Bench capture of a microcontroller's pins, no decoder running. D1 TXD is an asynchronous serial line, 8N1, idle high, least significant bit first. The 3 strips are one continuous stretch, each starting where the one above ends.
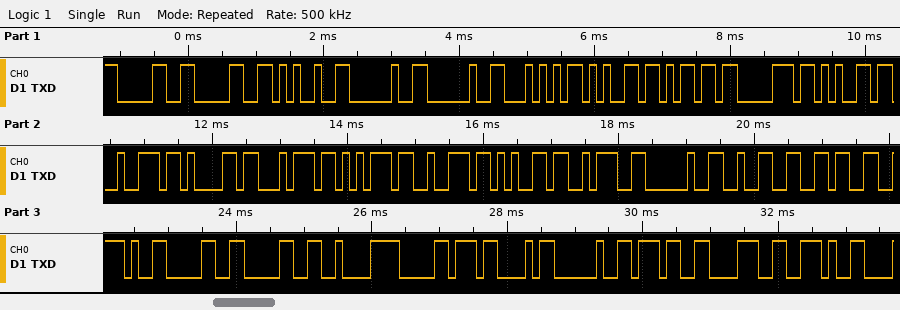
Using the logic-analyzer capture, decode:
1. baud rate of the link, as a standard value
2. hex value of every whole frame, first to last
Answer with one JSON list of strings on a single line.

["9600 baud", "0x30 0x30 0x25 0x20 0x20 0x54 0x65 0x6D 0x70 0x65 0x72 0x61 0x74 0x75 0x72 0x65 0x3A 0x20 0x32 0x36 0x2E 0x30 0x30 0xC2 0xB0 0x43 0x20 0x37 0x38 0x2E"]
